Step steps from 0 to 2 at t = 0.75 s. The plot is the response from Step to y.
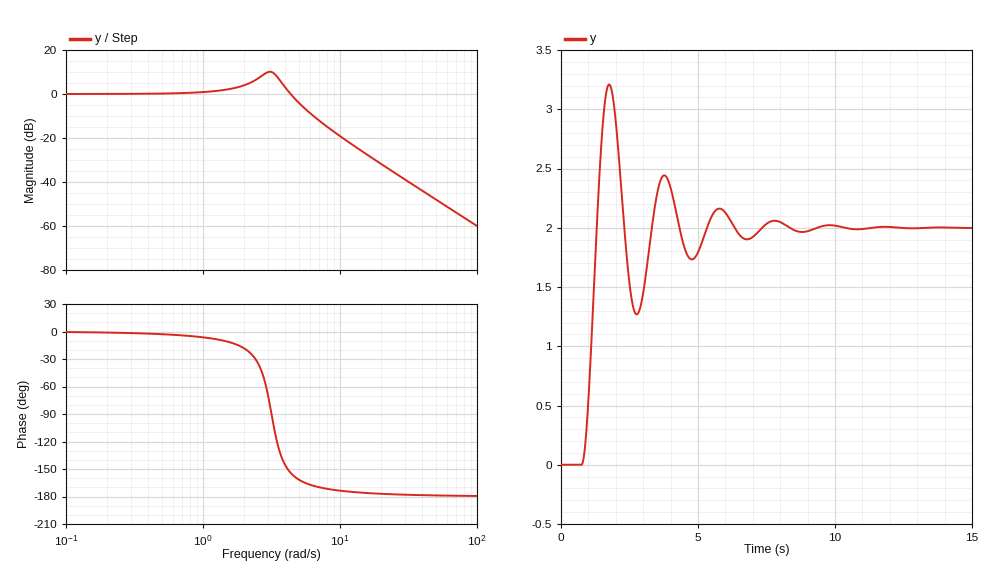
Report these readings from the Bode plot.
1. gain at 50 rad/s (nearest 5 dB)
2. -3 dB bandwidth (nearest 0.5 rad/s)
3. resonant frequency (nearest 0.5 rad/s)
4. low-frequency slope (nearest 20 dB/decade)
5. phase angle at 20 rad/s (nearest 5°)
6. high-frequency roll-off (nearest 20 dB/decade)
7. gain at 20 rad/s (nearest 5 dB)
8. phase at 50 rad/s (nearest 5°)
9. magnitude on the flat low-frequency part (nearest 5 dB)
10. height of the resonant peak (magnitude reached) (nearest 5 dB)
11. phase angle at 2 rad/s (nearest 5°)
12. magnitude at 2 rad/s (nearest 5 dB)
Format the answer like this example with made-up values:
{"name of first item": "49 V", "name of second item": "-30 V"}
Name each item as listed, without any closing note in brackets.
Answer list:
{"gain at 50 rad/s": "-50 dB", "-3 dB bandwidth": "5.0 rad/s", "resonant frequency": "3.0 rad/s", "low-frequency slope": "0 dB/decade", "phase angle at 20 rad/s": "-175°", "high-frequency roll-off": "-40 dB/decade", "gain at 20 rad/s": "-30 dB", "phase at 50 rad/s": "-180°", "magnitude on the flat low-frequency part": "0 dB", "height of the resonant peak (magnitude reached)": "10 dB", "phase angle at 2 rad/s": "-20°", "magnitude at 2 rad/s": "5 dB"}
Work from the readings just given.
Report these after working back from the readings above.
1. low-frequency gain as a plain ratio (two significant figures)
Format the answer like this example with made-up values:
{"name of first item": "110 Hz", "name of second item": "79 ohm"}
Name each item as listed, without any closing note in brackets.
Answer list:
{"low-frequency gain as a plain ratio": "1.0"}
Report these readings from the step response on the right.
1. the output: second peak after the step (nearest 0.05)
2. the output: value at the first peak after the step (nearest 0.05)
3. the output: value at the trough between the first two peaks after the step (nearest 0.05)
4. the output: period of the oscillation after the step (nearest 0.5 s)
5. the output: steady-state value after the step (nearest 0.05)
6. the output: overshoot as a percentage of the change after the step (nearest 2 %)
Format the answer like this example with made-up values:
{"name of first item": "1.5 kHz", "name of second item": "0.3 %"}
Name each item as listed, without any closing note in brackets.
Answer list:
{"the output: second peak after the step": "2.45", "the output: value at the first peak after the step": "3.20", "the output: value at the trough between the first two peaks after the step": "1.25", "the output: period of the oscillation after the step": "2.0 s", "the output: steady-state value after the step": "2.00", "the output: overshoot as a percentage of the change after the step": "60 %"}
